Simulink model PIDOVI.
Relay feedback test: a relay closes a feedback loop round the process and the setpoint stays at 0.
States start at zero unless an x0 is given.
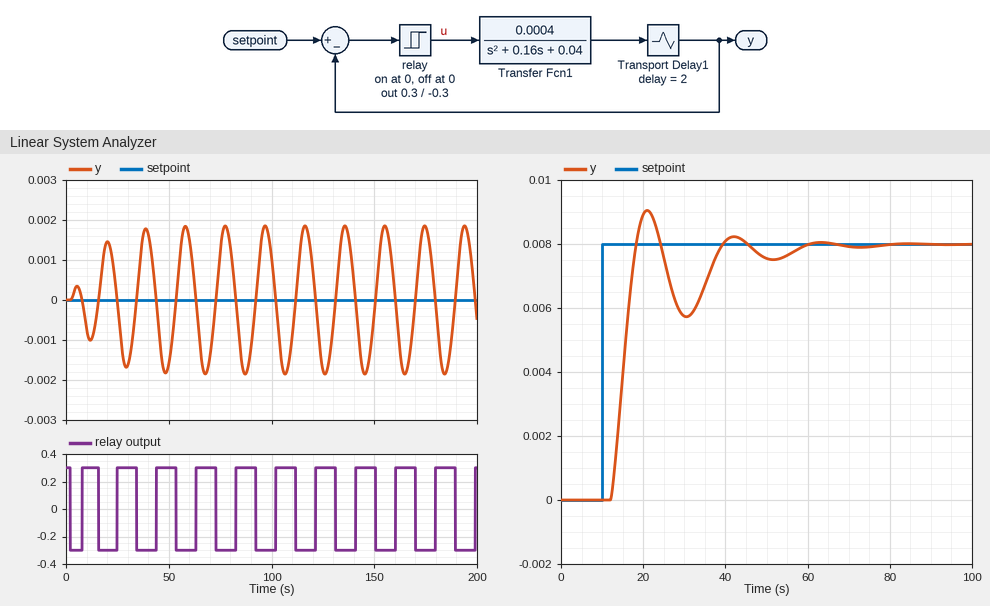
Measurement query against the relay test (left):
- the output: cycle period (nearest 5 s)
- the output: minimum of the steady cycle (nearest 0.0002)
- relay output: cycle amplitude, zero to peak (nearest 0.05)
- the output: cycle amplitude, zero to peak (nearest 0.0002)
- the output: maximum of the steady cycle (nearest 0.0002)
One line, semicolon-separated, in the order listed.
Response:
20 s; -0.0018; 0.30; 0.0018; 0.0018
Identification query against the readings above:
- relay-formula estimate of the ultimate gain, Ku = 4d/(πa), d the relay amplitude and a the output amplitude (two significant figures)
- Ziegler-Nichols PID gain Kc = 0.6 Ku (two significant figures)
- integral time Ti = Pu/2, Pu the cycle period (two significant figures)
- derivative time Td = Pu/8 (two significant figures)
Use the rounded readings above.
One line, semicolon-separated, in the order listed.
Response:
210; 130; 10 s; 2.5 s
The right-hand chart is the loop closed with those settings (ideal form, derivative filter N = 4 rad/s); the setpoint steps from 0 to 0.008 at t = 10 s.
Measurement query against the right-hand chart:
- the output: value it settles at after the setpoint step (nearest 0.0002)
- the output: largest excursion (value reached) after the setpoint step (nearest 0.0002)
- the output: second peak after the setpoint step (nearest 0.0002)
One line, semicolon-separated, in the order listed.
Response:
0.0080; 0.0090; 0.0082
